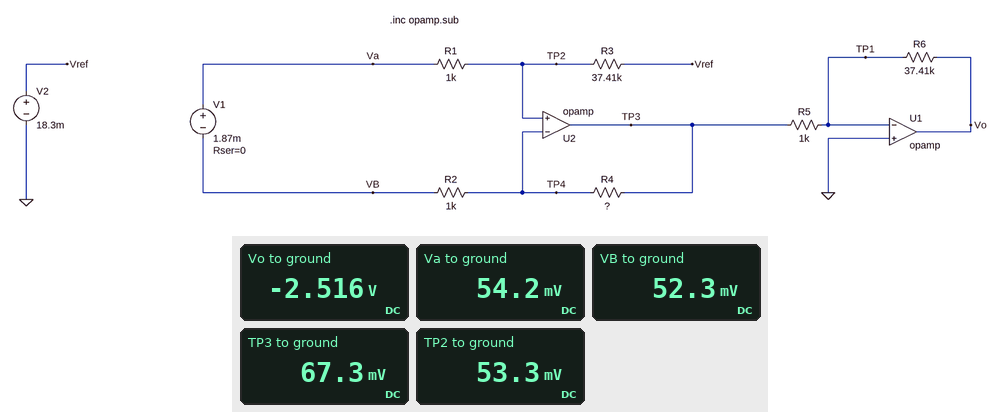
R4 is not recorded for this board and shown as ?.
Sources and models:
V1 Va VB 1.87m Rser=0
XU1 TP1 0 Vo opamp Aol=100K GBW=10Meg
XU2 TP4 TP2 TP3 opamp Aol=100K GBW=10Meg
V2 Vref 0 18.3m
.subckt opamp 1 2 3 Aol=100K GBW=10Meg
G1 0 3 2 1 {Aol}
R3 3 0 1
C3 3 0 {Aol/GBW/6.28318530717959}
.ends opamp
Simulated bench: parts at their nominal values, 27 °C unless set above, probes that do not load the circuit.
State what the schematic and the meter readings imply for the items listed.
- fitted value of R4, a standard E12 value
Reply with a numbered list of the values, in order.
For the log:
1. 15 kΩ
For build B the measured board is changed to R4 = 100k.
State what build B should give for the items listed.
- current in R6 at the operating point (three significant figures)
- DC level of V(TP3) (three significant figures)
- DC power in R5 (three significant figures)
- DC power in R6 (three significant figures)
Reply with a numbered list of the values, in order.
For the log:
1. 147 µA
2. 147 mV
3. 21.5 µW
4. 804 µW
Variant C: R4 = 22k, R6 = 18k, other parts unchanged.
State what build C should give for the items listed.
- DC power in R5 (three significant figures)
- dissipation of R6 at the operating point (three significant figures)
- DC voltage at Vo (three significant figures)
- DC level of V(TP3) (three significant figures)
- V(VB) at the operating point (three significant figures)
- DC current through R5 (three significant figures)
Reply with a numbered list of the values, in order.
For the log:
1. 5.45 µW
2. 98.1 µW
3. -1.33 V
4. 73.8 mV
5. 52.3 mV
6. 73.8 µA
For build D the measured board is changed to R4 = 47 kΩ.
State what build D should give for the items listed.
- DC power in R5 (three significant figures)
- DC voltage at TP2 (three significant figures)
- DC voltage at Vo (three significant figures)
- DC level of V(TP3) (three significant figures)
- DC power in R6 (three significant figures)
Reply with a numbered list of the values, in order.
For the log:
1. 9.44 µW
2. 53.3 mV
3. -3.63 V
4. 97.2 mV
5. 353 µW
